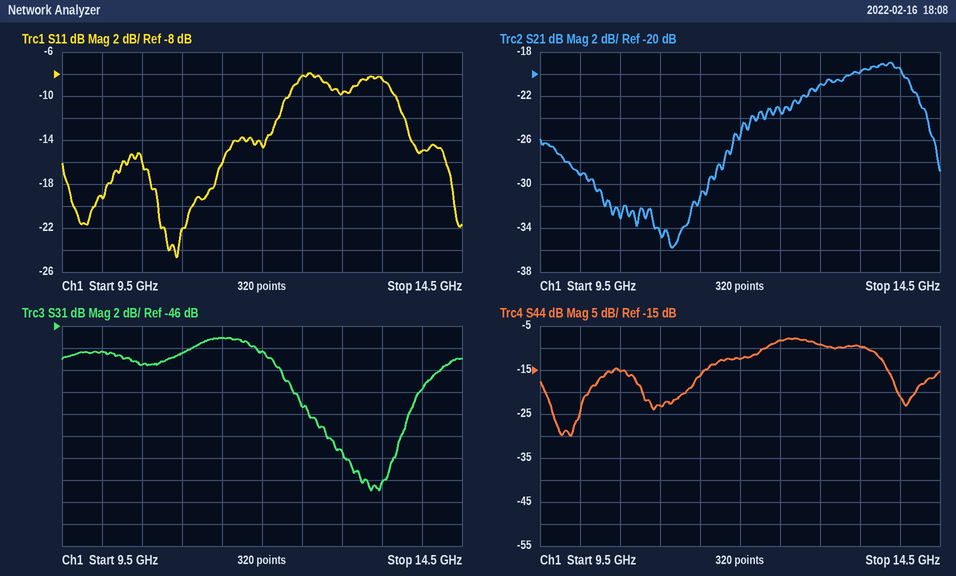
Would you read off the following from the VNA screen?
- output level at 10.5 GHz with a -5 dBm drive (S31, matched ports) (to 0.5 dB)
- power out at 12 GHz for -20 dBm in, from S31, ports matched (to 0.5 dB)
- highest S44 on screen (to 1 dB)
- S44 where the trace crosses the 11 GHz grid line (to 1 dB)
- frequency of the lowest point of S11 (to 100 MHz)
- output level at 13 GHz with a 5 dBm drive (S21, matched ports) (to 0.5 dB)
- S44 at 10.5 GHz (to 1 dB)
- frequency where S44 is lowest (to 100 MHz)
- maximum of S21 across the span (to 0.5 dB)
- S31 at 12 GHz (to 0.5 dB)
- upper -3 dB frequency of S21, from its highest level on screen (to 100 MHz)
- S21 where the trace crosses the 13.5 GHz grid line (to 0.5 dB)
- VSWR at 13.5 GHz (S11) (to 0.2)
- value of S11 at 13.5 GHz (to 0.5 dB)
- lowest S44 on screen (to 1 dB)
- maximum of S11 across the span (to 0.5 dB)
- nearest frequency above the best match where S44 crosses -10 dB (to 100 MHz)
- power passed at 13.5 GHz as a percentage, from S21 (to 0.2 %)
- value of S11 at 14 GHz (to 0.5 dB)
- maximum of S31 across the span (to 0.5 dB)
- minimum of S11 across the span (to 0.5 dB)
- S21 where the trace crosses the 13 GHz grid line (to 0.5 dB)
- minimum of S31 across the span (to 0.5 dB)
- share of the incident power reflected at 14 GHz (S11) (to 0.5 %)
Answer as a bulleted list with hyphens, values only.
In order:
- -54.5 dBm
- -68.5 dBm
- -8 dB
- -23 dB
- 10.9 GHz
- -16.0 dBm
- -15 dB
- 9.9 GHz
- -19.0 dB
- -48.5 dB
- 14.2 GHz
- -20.0 dB
- 2.2
- -8.5 dB
- -30 dB
- -8.0 dB
- 12.3 GHz
- 1.0 %
- -15.0 dB
- -47.0 dB
- -24.5 dB
- -21.0 dB
- -61.0 dB
- 3.0 %
